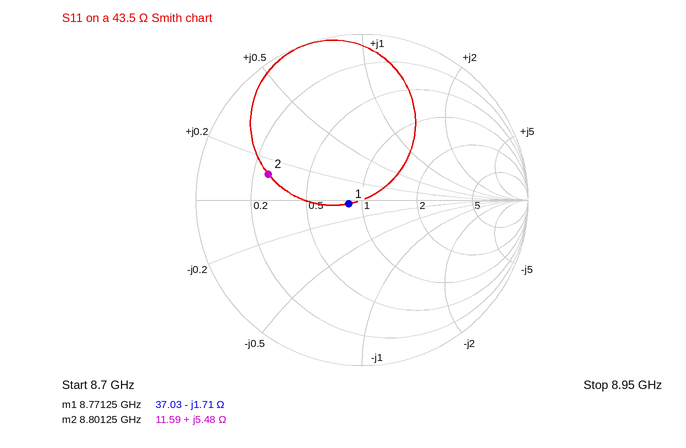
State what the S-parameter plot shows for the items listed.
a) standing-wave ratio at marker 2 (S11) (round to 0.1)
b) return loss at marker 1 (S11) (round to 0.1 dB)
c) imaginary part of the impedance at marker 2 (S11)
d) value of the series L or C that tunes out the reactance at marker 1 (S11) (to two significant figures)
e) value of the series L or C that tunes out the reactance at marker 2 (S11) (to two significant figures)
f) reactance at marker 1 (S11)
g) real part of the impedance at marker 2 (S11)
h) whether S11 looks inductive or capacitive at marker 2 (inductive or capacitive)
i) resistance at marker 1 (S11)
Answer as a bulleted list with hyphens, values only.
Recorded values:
- 3.8
- 21.6 dB
- +5.48 Ω
- 31 pH
- 3.3 pF
- -1.71 Ω
- 11.59 Ω
- inductive
- 37.03 Ω
